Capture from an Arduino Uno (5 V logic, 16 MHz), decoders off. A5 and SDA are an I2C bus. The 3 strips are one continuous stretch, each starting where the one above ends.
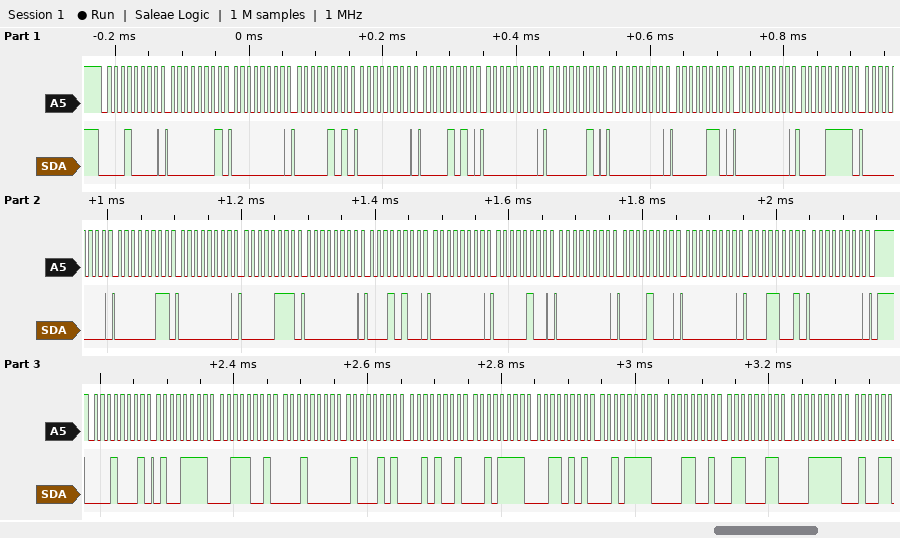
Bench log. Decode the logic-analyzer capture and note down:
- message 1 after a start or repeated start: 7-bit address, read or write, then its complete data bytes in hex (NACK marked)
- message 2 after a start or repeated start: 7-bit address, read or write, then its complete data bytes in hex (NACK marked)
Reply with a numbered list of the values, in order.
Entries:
1. 0x08 write: 01 00 05 00 0A 00 02 00 06 00 0F 00 03 00 07 00 14 00 04 00 08 00 19 00
2. 0x08 read: 4F 39 10 45 29 2F 35 2F 19 63 1F
